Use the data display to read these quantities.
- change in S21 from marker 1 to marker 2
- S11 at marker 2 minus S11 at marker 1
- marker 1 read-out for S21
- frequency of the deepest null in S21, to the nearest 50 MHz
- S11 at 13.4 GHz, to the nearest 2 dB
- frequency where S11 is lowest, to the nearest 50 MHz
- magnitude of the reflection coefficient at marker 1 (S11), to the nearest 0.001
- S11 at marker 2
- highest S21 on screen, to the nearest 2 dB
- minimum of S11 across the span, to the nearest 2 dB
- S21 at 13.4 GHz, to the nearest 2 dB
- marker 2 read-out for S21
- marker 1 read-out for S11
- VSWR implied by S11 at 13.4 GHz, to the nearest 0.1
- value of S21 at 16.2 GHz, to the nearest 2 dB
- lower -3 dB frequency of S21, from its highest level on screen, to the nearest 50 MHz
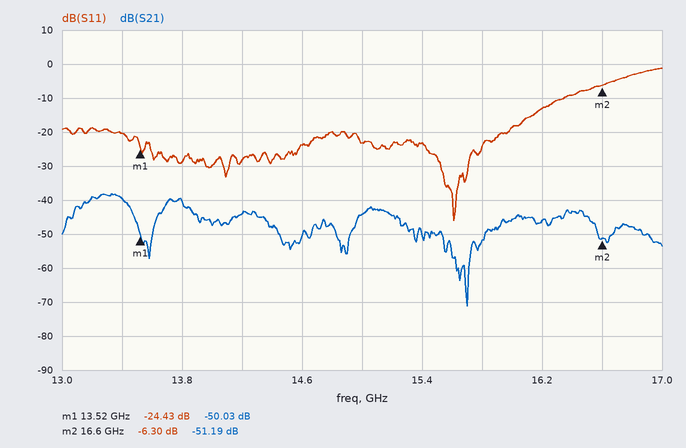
-1.16 dB
18.13 dB
-50.03 dB
15.70 GHz
-20 dB
15.60 GHz
0.060
-6.30 dB
-38 dB
-46 dB
-40 dB
-51.19 dB
-24.43 dB
1.2
-46 dB
13.15 GHz
